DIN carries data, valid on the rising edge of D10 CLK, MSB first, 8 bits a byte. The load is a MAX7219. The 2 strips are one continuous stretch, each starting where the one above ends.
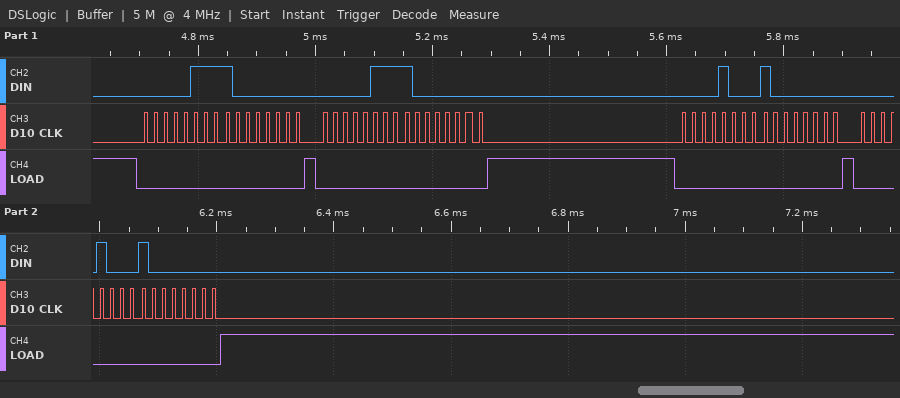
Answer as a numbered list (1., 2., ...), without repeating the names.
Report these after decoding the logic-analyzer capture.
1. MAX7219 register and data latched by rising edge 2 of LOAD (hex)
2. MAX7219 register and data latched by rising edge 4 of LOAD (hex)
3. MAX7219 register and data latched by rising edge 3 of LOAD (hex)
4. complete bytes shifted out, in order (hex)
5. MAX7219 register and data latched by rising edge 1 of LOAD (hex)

1. register 0x7, data 0x80
2. register 0x8, data 0x80
3. register 0x8, data 0x80
4. 07 80 07 80 08 80 08 80
5. register 0x7, data 0x80
